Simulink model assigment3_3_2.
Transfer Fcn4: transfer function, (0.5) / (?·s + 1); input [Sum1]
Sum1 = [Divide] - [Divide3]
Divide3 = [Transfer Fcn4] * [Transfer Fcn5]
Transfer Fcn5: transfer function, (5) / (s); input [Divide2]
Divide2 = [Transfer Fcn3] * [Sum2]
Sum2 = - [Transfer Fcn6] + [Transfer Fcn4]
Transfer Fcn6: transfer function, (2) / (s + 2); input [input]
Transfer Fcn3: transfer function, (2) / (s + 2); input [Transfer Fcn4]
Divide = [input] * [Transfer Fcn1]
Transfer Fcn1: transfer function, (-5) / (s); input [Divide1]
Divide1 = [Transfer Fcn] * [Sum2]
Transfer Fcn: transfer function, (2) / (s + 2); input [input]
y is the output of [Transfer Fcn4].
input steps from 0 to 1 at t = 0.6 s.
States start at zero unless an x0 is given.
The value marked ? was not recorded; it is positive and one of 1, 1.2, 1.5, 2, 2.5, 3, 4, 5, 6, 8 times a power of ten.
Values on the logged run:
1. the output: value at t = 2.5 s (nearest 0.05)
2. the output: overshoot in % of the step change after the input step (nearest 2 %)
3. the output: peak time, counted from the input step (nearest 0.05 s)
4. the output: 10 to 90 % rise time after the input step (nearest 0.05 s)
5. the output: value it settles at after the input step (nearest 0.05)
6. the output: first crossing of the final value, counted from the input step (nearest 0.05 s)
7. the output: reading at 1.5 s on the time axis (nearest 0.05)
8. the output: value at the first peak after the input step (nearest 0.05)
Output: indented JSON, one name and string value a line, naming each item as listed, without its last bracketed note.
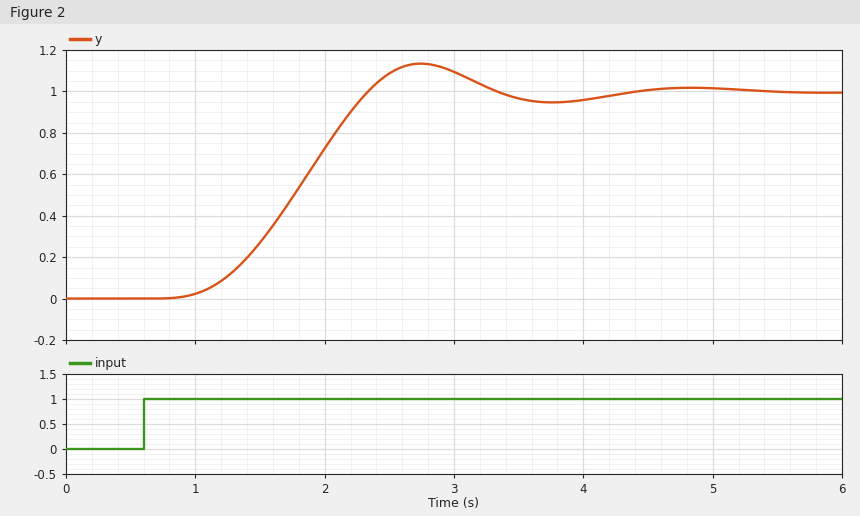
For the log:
{
  "the output: value at t = 2.5 s": "1.10",
  "the output: overshoot in % of the step change after the input step": "14 %",
  "the output: peak time, counted from the input step": "2.15 s",
  "the output: 10 to 90 % rise time after the input step": "0.95 s",
  "the output: value it settles at after the input step": "1.00",
  "the output: first crossing of the final value, counted from the input step": "1.75 s",
  "the output: reading at 1.5 s on the time axis": "0.25",
  "the output: value at the first peak after the input step": "1.15"
}
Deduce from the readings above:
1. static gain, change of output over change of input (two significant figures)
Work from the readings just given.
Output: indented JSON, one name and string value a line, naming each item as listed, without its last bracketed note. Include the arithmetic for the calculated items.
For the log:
{
  "static gain, change of output over change of input": "(1 - 0) / (1 - 0) = 1.0"
}
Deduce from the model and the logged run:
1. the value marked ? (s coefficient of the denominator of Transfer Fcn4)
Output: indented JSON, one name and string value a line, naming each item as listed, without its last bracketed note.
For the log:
{
  "the value marked ?": "0.5"
}
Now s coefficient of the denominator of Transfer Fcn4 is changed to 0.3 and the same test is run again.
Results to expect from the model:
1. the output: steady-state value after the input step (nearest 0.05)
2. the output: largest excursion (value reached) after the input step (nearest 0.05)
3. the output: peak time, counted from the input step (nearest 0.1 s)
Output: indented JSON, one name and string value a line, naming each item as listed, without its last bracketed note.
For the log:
{
  "the output: steady-state value after the input step": "1.00",
  "the output: largest excursion (value reached) after the input step": "1.05",
  "the output: peak time, counted from the input step": "2.0 s"
}
